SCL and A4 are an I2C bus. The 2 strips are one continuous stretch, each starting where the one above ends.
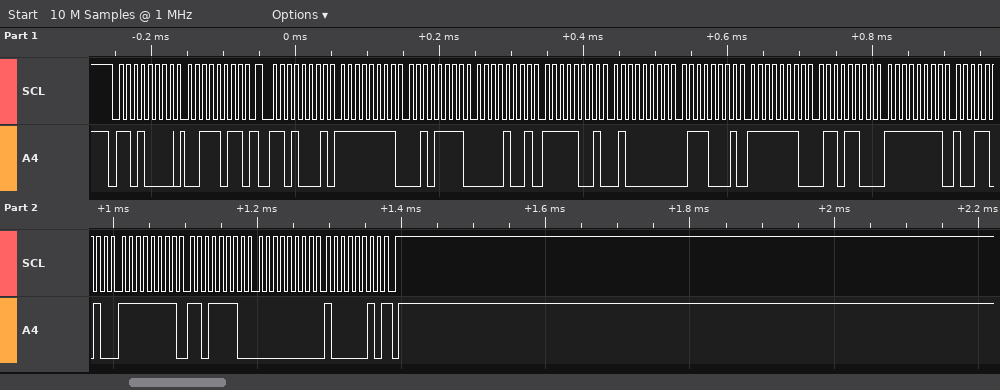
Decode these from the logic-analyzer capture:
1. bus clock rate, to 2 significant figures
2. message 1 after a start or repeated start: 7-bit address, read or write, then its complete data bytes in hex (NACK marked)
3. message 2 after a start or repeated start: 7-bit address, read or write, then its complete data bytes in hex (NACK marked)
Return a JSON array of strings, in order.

["100 kHz", "0x68 write: 3B", "0x68 read: FF 2F 09 F9 40 71 FE 6C FF 9A FF DE 00 82 NACK"]
